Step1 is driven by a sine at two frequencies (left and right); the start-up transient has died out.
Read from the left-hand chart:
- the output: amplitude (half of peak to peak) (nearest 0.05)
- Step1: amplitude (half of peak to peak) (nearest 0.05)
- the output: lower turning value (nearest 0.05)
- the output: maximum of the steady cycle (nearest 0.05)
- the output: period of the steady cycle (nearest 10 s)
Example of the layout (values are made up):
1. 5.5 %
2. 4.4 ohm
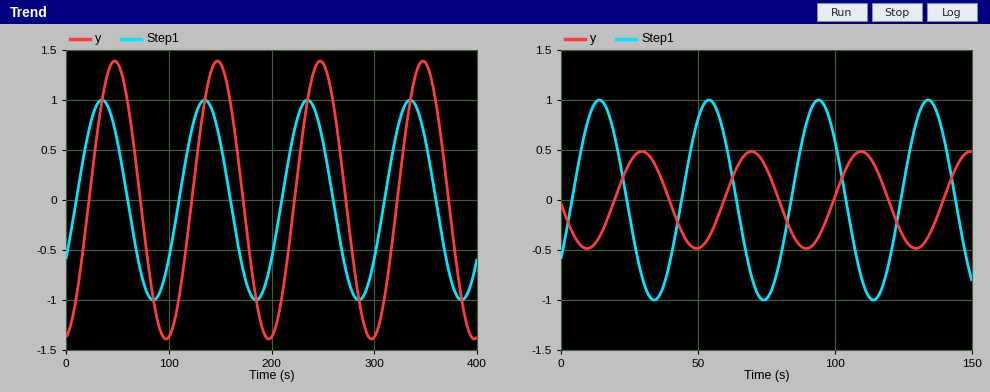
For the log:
1. 1.40
2. 1.00
3. -1.40
4. 1.40
5. 100 s
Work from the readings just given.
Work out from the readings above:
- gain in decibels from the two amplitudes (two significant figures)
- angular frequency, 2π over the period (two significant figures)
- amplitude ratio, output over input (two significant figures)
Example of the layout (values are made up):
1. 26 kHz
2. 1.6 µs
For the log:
1. 2.9 dB
2. 0.063 rad/s
3. 1.4
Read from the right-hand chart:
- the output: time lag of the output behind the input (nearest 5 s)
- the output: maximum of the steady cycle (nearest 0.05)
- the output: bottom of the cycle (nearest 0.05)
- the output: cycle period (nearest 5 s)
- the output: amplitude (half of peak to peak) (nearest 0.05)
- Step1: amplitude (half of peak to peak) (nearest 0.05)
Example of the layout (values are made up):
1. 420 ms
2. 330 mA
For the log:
1. 15 s
2. 0.50
3. -0.50
4. 40 s
5. 0.50
6. 1.00
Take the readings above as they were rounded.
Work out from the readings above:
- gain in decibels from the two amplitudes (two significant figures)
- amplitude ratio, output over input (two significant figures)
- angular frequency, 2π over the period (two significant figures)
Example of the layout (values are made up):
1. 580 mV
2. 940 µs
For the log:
1. -6.0 dB
2. 0.50
3. 0.16 rad/s
